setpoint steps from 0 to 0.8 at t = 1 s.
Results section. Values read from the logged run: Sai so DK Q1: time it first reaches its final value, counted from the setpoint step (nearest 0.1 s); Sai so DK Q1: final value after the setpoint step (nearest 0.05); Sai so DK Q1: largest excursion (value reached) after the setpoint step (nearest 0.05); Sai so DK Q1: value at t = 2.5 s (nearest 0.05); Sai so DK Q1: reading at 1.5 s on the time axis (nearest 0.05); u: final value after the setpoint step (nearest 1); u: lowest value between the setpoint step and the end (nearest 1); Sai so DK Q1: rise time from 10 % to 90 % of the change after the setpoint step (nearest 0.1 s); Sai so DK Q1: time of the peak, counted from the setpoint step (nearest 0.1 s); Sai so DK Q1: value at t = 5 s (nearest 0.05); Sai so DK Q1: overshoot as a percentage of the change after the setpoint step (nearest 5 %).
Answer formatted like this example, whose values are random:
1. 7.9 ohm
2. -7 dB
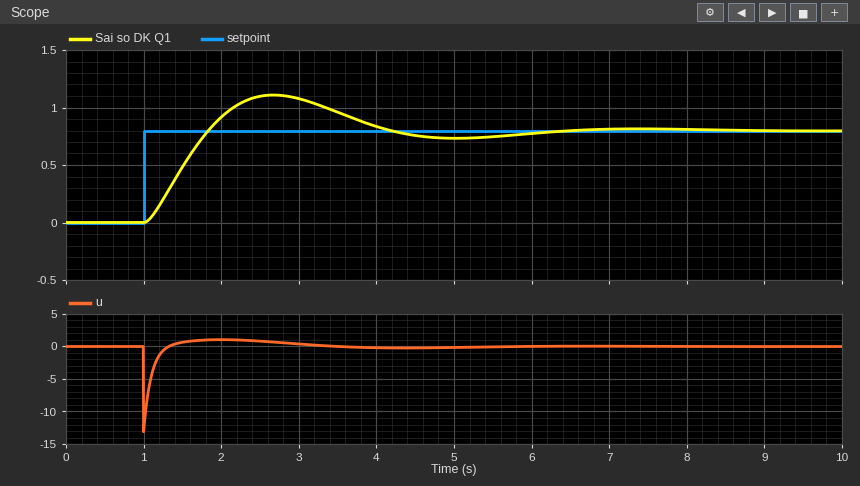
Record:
1. 0.8 s
2. 0.80
3. 1.10
4. 1.10
5. 0.50
6. 0
7. -13
8. 0.6 s
9. 1.7 s
10. 0.75
11. 40 %
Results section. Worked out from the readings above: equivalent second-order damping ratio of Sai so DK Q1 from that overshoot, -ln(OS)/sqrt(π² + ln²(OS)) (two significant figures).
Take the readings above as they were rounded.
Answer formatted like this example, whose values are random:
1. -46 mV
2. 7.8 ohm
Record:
1. 0.28
